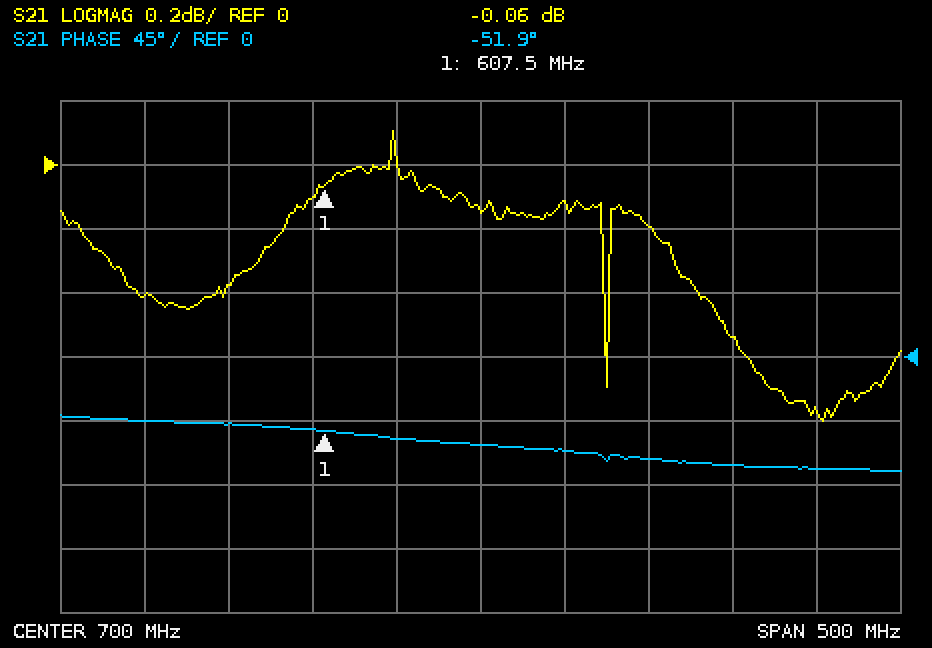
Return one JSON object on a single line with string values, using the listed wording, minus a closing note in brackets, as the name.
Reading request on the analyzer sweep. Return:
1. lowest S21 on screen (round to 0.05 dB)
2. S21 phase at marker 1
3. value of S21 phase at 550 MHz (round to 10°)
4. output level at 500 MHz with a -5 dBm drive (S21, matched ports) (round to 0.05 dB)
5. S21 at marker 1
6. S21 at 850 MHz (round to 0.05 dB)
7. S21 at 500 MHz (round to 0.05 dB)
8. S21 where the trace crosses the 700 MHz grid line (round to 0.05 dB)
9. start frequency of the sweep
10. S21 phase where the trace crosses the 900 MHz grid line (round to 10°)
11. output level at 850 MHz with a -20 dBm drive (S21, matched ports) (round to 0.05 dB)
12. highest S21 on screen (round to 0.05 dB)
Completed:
{"lowest S21 on screen": "-0.80 dB", "S21 phase at marker 1": "-51.9°", "value of S21 phase at 550 MHz": "-50°", "output level at 500 MHz with a -5 dBm drive (S21, matched ports)": "-5.40 dBm", "S21 at marker 1": "-0.06 dB", "S21 at 850 MHz": "-0.55 dB", "S21 at 500 MHz": "-0.40 dB", "S21 where the trace crosses the 700 MHz grid line": "-0.15 dB", "start frequency of the sweep": "450 MHz", "S21 phase where the trace crosses the 900 MHz grid line": "-80°", "output level at 850 MHz with a -20 dBm drive (S21, matched ports)": "-20.55 dBm", "highest S21 on screen": "0.10 dB"}
